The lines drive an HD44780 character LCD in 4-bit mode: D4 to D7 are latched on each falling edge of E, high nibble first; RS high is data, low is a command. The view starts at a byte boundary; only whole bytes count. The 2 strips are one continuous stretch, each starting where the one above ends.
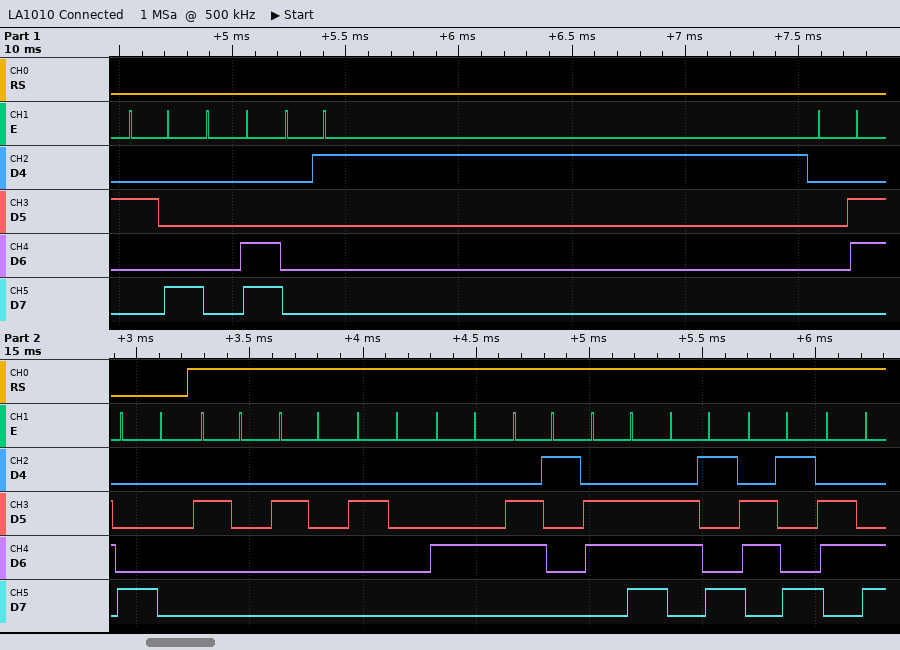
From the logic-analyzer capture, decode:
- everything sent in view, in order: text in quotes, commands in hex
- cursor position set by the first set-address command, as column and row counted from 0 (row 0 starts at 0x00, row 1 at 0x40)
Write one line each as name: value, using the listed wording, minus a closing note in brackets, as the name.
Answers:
everything sent in view, in order: text in quotes, commands in hex: 0x28 0x0C 0x01 0x06 0x80 "   Daniil"
cursor position set by the first set-address command, as column and row counted from 0: column 0, row 0
